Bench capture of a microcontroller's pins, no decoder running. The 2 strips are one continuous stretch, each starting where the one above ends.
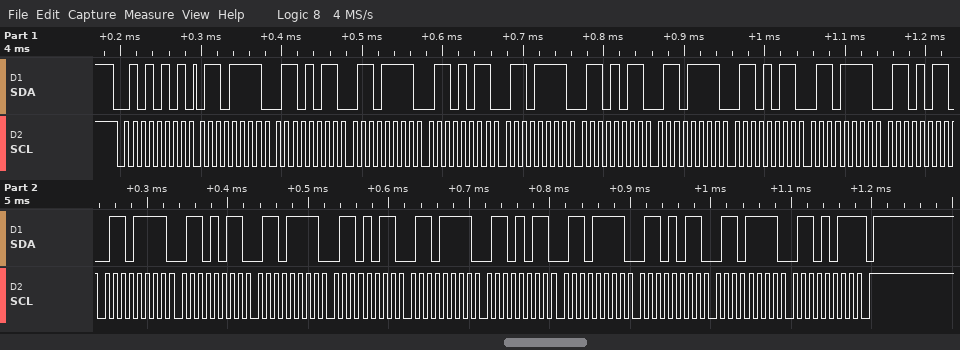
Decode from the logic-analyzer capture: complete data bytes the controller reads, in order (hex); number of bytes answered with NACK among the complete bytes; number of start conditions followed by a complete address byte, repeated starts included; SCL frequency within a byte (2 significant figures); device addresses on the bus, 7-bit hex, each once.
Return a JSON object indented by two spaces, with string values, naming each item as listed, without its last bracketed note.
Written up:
{
  "complete data bytes the controller reads, in order": "6F 6B 6F 6B 6F 6B 6F 6B 6F 6B 6F 6B 6F 6B 6F 6B 6F 6B 6F 6B",
  "number of bytes answered with NACK among the complete bytes": "1",
  "number of start conditions followed by a complete address byte, repeated starts included": "1",
  "SCL frequency within a byte": "100 kHz",
  "device addresses on the bus, 7-bit hex, each once": "0x2A"
}
